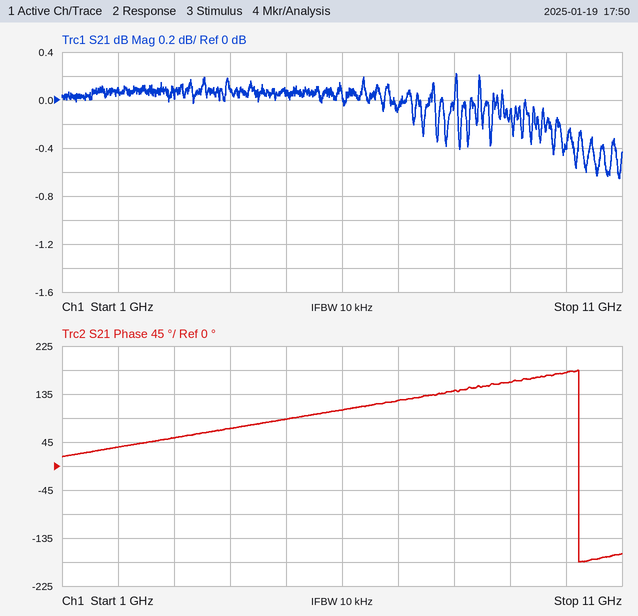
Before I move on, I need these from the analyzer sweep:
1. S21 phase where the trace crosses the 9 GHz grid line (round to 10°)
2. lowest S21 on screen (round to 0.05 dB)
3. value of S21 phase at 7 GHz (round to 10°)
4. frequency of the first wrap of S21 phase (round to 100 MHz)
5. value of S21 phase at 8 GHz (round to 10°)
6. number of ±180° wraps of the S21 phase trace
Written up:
160°
-0.65 dB
120°
10.2 GHz
140°
1
